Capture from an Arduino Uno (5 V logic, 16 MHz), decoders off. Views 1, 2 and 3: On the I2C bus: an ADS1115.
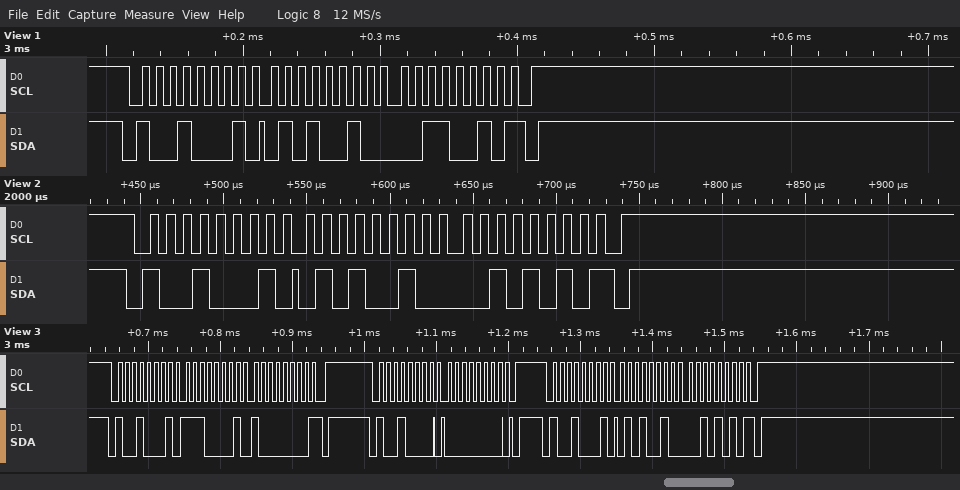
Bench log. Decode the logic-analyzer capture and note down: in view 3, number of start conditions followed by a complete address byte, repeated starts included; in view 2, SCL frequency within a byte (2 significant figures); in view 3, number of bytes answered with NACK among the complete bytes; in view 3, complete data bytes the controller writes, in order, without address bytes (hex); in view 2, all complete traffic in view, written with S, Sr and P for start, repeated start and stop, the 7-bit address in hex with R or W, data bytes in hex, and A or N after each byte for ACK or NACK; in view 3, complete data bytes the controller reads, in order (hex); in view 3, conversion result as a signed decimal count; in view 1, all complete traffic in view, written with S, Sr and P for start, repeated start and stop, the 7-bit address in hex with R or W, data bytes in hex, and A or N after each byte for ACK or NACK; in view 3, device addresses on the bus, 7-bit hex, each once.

3
100 kHz
2
00
S 48R A 52 A 2A N P
E1 80 52 2A
21034
S 48R A 52 A 32 N P
0x48
